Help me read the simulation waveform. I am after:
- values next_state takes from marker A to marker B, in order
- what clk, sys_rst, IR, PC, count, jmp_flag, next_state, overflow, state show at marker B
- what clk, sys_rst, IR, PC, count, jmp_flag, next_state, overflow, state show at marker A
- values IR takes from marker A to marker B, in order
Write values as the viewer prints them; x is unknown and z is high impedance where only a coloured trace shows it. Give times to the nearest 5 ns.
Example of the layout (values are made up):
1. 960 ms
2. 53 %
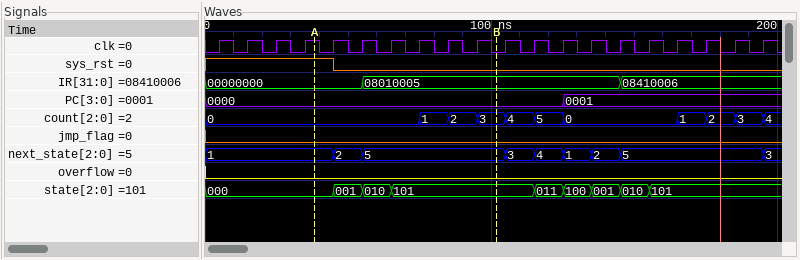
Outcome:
1. 1, 2, 5
2. clk=0, sys_rst=0, IR=08010005, PC=0000, count=3, jmp_flag=0, next_state=5, overflow=0, state=101
3. clk=1, sys_rst=1, IR=00000000, PC=0000, count=0, jmp_flag=0, next_state=1, overflow=0, state=000
4. 00000000, 08010005
